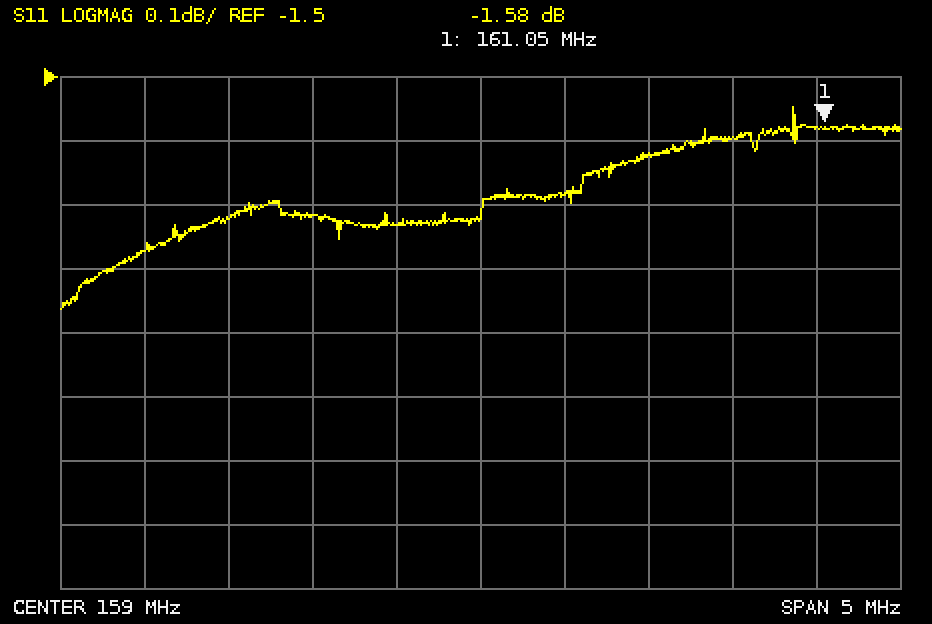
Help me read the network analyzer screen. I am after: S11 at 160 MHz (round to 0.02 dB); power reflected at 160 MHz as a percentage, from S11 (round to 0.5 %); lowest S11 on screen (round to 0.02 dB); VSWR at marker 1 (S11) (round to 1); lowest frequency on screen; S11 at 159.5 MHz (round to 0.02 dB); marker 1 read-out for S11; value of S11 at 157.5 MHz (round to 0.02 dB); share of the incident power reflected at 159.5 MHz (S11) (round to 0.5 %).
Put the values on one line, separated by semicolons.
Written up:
-1.62 dB; 69.0 %; -1.86 dB; 11; 156.5 MHz; -1.68 dB; -1.58 dB; -1.72 dB; 68.0 %
